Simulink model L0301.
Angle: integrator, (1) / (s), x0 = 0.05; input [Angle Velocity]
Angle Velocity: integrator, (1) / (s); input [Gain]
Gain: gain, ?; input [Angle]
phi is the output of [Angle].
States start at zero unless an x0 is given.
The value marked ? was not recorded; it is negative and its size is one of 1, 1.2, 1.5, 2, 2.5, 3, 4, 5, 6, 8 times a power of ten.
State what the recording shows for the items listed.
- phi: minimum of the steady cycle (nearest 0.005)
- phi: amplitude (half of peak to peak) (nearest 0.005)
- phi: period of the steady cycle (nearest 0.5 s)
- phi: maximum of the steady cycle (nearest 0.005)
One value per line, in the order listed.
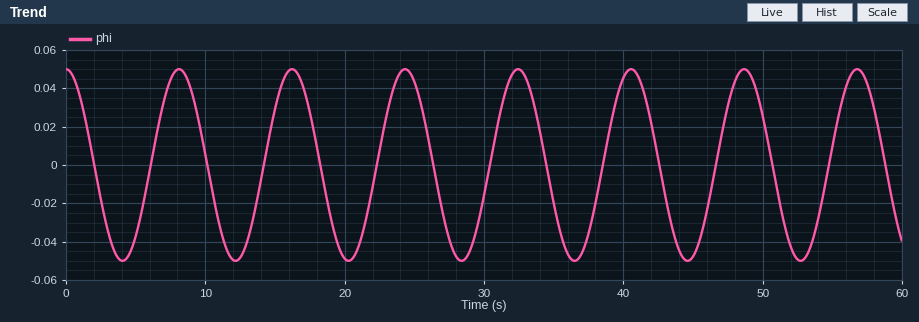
-0.050
0.050
8.0 s
0.050
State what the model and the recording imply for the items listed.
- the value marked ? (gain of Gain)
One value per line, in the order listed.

-0.6
